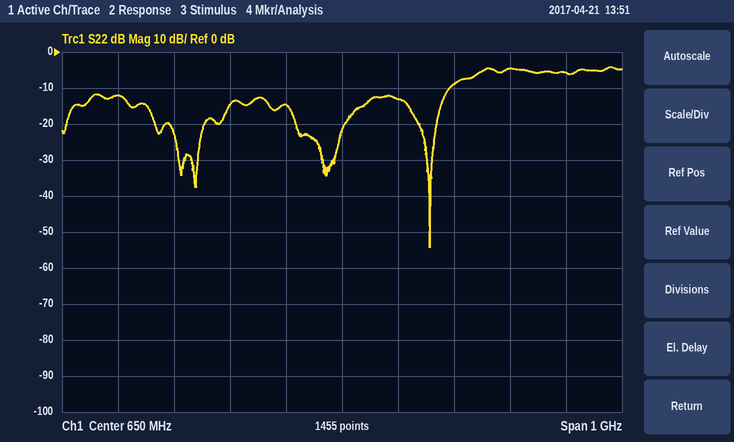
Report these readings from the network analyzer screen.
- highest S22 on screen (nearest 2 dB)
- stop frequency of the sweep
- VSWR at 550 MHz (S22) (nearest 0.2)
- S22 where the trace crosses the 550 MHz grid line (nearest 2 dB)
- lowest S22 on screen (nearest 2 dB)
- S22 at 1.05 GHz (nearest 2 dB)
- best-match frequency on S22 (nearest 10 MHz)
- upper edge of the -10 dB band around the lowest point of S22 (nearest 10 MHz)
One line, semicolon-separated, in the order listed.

-4 dB; 1.15 GHz; 1.4; -14 dB; -54 dB; -6 dB; 810 MHz; 840 MHz
